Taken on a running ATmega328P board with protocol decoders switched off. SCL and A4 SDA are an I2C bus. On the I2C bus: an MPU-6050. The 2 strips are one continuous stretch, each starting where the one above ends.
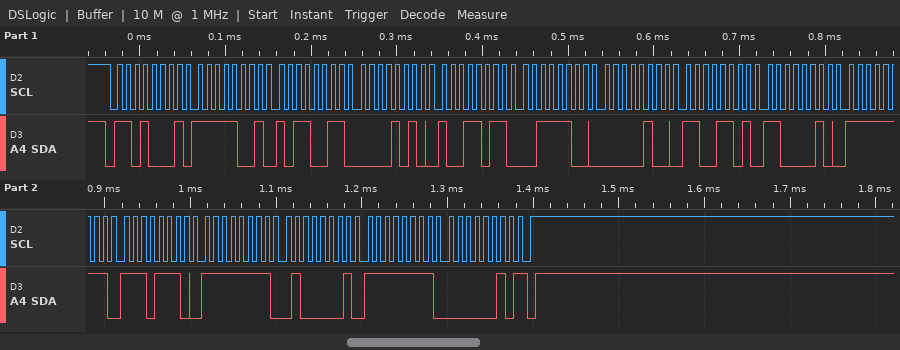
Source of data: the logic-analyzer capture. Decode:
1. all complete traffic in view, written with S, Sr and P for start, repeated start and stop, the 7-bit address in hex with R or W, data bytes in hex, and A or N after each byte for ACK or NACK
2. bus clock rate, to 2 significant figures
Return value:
S 68R A F9 A B3 A 0A A 9B A 3C A 04 A CD A C2 A FF A EE A FF A 41 A FF A 02 N P
100 kHz
